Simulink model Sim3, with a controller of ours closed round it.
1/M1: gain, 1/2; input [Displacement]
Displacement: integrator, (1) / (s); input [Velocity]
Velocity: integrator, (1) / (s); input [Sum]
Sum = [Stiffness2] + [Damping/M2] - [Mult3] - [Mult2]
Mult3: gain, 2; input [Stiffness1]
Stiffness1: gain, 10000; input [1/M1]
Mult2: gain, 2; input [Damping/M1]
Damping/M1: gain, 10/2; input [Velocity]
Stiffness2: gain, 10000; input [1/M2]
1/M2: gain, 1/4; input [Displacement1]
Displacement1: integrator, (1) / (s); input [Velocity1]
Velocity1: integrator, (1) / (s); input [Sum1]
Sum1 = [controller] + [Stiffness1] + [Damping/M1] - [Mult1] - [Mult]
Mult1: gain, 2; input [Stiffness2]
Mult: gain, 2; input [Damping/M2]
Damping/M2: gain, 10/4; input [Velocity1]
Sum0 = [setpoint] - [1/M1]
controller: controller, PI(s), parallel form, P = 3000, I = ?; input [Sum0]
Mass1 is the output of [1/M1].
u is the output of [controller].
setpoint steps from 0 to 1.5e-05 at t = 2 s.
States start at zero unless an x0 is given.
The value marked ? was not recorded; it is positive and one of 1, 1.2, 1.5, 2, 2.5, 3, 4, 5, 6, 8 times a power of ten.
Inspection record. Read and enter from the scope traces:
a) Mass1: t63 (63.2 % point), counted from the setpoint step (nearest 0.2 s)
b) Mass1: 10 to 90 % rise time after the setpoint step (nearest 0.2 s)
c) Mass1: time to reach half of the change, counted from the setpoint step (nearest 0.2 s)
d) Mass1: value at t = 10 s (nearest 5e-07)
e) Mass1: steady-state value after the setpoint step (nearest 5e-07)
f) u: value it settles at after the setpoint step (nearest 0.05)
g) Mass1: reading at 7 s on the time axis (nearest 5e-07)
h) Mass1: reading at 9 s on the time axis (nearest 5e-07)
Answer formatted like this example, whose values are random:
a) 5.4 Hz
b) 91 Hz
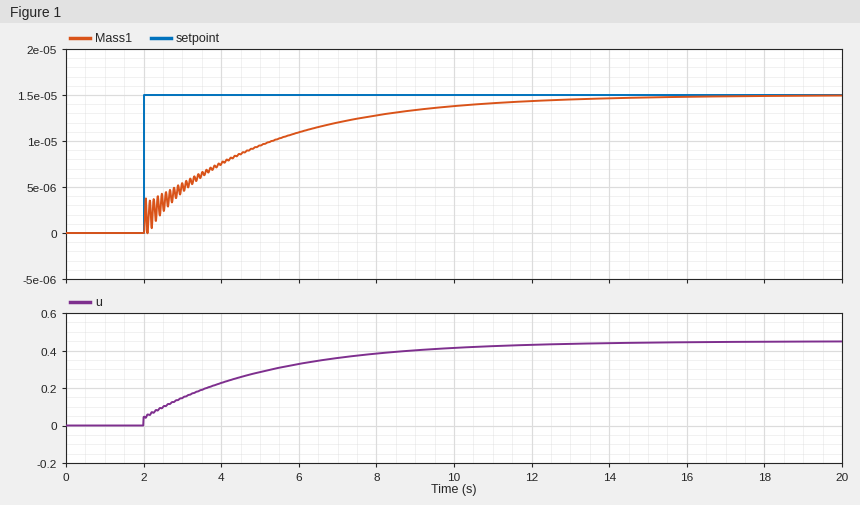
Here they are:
a) 3.0 s
b) 7.2 s
c) 2.0 s
d) 0.0000140
e) 0.0000150
f) 0.45
g) 0.0000120
h) 0.0000135
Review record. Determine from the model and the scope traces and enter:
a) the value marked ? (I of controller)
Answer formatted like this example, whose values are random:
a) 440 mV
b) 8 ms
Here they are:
a) 10000
